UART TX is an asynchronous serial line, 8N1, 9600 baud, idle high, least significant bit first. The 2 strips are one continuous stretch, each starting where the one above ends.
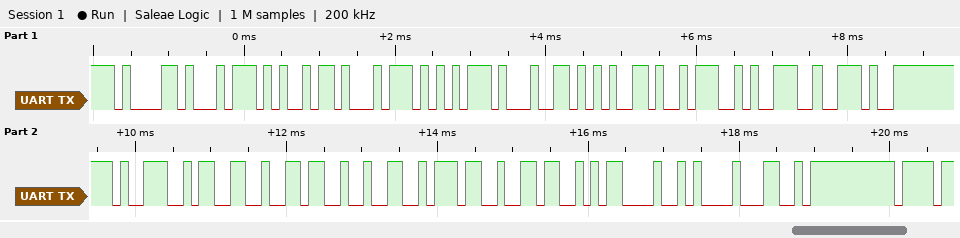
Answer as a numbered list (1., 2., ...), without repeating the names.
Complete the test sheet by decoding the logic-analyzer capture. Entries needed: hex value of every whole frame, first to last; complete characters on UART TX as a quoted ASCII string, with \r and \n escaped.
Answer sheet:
1. 61 74 69 74 75 64 65 3A 39 2E 39 33 36 32 37 36 0D 0A 4C
2. "atitude:9.936276\r\nL"
